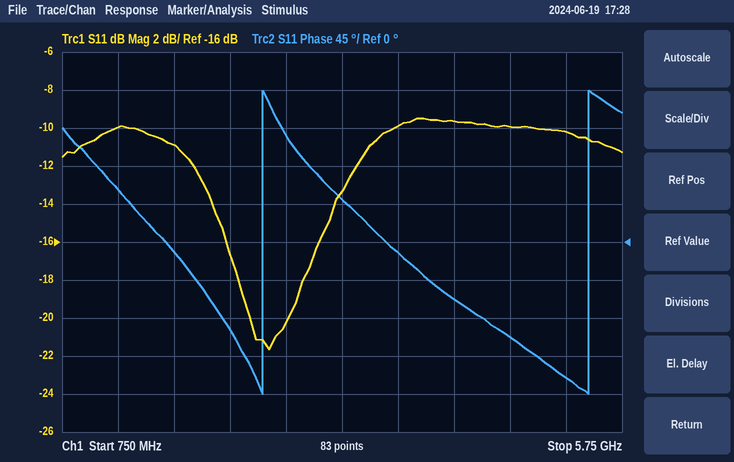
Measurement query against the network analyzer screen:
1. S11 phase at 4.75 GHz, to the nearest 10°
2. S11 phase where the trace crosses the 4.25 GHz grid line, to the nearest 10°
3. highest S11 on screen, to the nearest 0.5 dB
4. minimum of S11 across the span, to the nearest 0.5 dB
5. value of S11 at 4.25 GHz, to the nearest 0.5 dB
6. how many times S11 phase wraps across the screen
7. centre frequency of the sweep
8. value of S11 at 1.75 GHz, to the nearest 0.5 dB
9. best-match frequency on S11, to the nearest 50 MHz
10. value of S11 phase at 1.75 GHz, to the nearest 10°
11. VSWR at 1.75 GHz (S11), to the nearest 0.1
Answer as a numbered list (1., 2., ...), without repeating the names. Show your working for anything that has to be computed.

1. -110°
2. -70°
3. -9.5 dB
4. -21.5 dB
5. -9.5 dB
6. 2
7. 3.25 GHz
8. -11.0 dB
9. 2.60 GHz
10. -10°
11. |Γ| = 10^(-11/20) = 0.2818; VSWR = (1 + 0.2818)/(1 − 0.2818) ≈ 1.8
